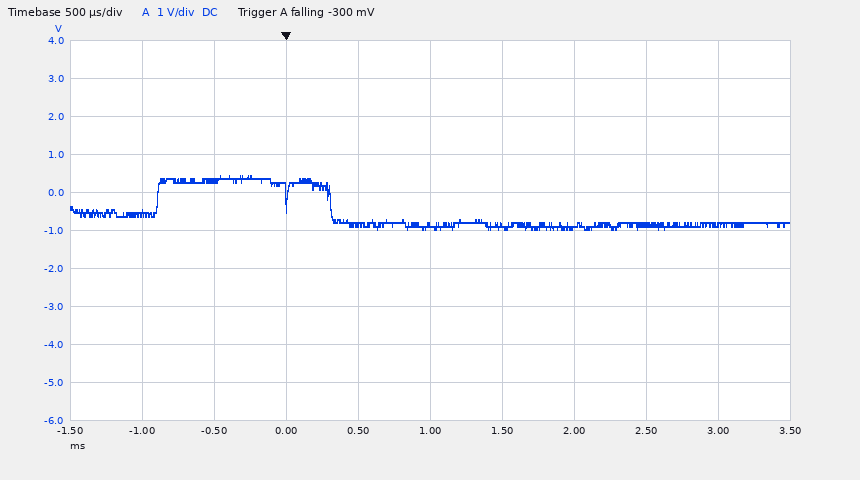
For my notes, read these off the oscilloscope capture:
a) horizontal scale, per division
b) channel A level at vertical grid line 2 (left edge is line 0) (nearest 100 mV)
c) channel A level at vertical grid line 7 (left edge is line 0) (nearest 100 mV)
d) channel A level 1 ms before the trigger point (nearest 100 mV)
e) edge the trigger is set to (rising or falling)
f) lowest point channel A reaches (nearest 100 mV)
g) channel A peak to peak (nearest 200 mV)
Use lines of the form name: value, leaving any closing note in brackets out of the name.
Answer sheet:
horizontal scale, per division: 500 µs
channel A level at vertical grid line 2 (left edge is line 0): 300 mV
channel A level at vertical grid line 7 (left edge is line 0): -900 mV
channel A level 1 ms before the trigger point: -500 mV
edge the trigger is set to: falling
lowest point channel A reaches: -1.0 V
channel A peak to peak: 1.4 V
